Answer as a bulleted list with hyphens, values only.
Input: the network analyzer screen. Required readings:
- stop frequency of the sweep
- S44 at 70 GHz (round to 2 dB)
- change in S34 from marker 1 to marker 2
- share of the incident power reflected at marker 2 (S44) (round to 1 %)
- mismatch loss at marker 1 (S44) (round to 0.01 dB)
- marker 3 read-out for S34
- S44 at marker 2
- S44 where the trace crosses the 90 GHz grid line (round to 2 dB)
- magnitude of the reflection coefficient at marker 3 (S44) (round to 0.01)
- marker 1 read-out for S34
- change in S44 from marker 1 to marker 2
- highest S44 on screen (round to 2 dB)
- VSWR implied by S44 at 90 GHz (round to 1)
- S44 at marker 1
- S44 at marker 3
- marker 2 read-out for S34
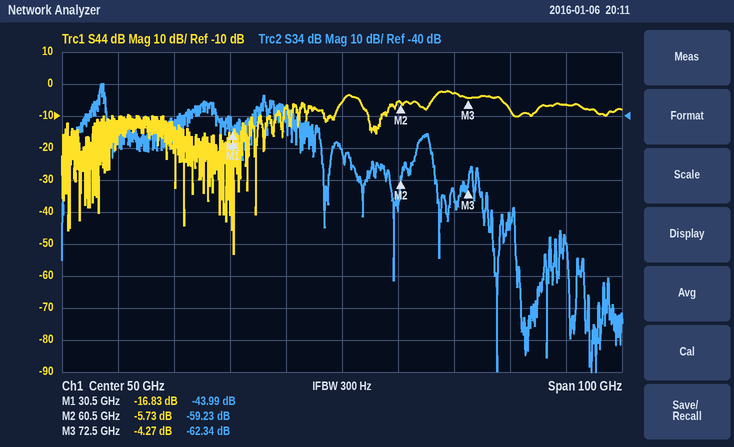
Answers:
- 100 GHz
- -2 dB
- -15.24 dB
- 27 %
- 0.09 dB
- -62.34 dB
- -5.73 dB
- -6 dB
- 0.61
- -43.99 dB
- 11.10 dB
- -2 dB
- 3
- -16.83 dB
- -4.27 dB
- -59.23 dB
